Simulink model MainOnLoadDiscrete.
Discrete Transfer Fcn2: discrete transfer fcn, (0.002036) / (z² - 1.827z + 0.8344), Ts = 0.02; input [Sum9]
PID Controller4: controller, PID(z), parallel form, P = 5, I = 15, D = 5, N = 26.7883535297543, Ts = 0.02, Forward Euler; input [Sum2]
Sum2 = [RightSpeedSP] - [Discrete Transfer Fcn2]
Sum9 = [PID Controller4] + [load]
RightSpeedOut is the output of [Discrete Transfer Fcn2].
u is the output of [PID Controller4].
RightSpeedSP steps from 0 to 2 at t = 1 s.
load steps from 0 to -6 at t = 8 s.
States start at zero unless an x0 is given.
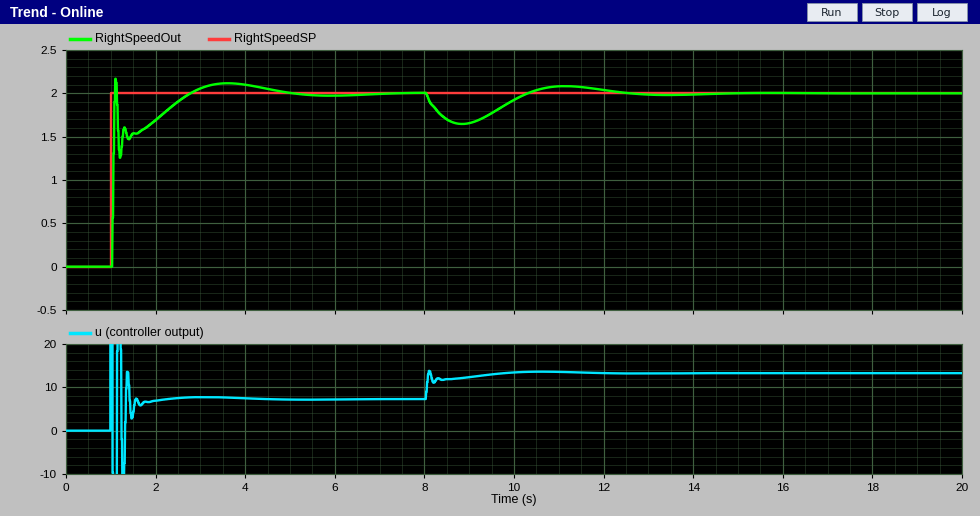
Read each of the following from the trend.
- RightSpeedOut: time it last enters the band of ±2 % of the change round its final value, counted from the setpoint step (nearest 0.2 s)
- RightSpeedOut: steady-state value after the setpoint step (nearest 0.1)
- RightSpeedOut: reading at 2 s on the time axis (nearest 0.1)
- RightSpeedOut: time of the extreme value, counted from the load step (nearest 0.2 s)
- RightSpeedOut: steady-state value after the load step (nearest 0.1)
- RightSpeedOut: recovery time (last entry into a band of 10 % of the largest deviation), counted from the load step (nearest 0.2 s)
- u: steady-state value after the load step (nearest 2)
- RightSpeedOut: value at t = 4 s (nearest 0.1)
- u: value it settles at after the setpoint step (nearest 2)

3.6 s
2.0
1.7
0.8 s
2.0
4.0 s
14
2.1
8
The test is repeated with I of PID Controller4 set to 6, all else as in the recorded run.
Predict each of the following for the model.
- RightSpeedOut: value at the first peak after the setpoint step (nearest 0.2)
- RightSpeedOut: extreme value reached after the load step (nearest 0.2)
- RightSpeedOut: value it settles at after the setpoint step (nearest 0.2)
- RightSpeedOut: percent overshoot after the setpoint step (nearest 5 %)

2.2
1.6
2.0
10 %
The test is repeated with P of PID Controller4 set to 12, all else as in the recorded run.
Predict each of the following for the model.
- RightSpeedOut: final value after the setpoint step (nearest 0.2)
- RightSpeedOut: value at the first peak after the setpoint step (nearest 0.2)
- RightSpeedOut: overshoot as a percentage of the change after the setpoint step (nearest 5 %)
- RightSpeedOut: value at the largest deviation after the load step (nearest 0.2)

2.0
2.4
15 %
1.8
